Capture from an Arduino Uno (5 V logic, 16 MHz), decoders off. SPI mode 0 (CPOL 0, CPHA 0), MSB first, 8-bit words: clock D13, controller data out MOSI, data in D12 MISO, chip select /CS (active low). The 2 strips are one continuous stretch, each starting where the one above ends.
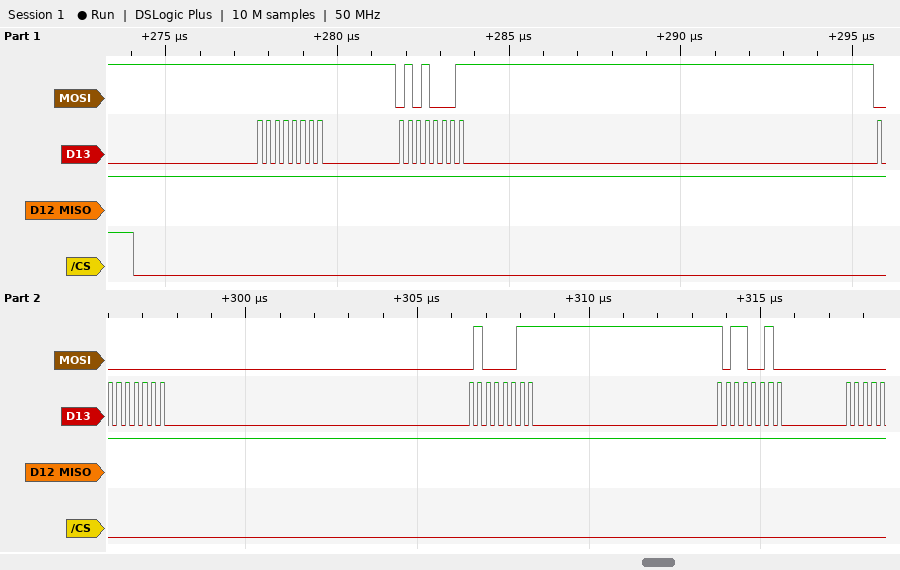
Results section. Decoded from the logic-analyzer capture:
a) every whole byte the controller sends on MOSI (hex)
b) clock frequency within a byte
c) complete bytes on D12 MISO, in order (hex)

0xFF 0x51 0x00 0x43 0xB2
4 MHz
0xFF 0xFF 0xFF 0xFF 0xFF
